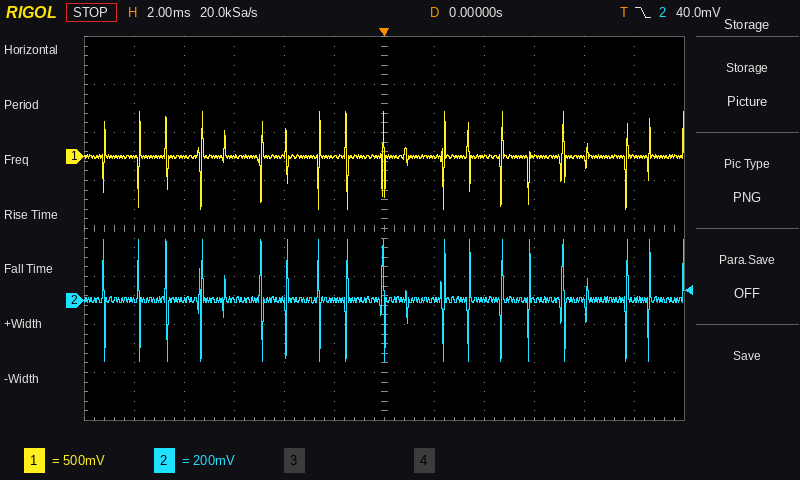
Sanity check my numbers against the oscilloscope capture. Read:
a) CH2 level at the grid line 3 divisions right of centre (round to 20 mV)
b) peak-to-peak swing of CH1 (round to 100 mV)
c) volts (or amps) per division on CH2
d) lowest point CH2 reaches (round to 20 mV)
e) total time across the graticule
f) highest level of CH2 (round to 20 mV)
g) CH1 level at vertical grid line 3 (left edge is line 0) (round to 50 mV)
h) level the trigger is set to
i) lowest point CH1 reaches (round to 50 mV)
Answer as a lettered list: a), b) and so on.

a) 0 mV
b) 1.00 V
c) 200 mV
d) -260 mV
e) 24 ms
f) 260 mV
g) 0 mV
h) 40.0 mV
i) -550 mV
